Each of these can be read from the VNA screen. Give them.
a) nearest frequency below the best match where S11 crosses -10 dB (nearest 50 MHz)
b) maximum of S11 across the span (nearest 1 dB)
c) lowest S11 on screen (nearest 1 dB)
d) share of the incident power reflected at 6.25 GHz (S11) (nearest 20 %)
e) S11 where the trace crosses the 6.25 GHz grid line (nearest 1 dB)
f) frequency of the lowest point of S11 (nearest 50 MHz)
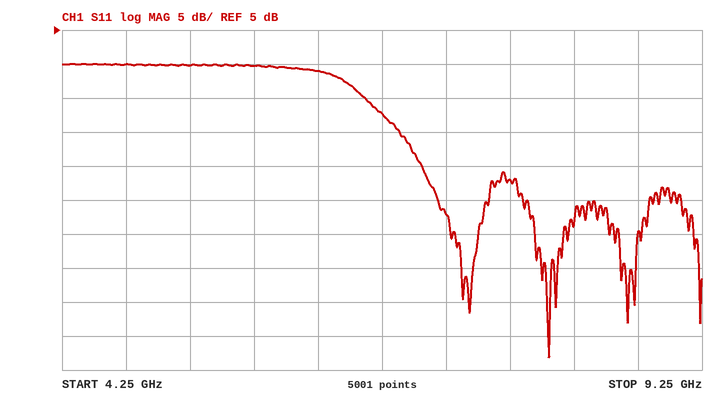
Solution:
6.90 GHz
0 dB
-43 dB
80 %
-1 dB
8.05 GHz
